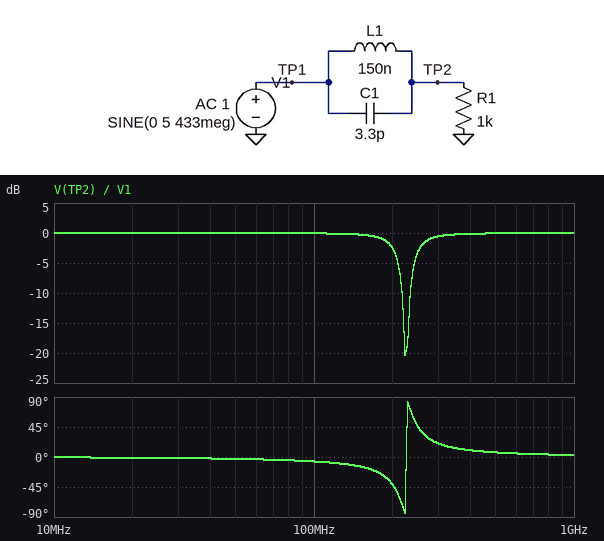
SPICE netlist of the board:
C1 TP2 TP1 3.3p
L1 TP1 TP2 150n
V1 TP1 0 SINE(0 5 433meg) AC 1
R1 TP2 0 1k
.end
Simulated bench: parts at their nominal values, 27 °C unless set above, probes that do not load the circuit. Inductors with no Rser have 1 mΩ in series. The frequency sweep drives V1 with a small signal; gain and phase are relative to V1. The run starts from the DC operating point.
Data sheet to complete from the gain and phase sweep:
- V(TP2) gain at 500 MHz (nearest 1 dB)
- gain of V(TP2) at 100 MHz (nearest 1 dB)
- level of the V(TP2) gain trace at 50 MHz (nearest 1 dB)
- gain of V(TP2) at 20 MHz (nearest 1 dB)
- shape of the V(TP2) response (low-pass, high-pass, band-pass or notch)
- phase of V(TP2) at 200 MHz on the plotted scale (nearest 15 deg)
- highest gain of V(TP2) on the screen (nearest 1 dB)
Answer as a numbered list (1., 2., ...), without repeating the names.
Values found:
1. 0 dB
2. 0 dB
3. 0 dB
4. 0 dB
5. notch
6. -45 deg
7. 0 dB
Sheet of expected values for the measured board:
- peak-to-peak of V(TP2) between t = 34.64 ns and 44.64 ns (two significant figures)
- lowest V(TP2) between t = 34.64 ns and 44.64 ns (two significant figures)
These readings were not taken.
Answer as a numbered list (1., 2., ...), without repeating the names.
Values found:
1. 9.9 V
2. -4.9 V
